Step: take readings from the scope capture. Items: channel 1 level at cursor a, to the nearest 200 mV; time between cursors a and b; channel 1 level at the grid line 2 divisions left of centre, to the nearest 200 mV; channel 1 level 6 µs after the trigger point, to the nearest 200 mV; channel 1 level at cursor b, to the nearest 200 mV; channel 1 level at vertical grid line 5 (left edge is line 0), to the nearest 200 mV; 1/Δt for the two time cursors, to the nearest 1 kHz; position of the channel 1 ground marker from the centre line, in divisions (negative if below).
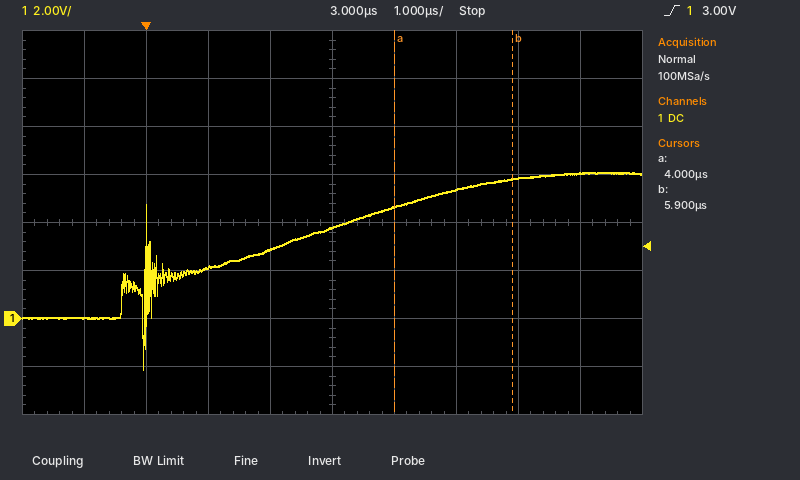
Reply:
4.6 V
1.9 µs
2.2 V
5.8 V
5.8 V
3.8 V
526 kHz
-2.0 div
